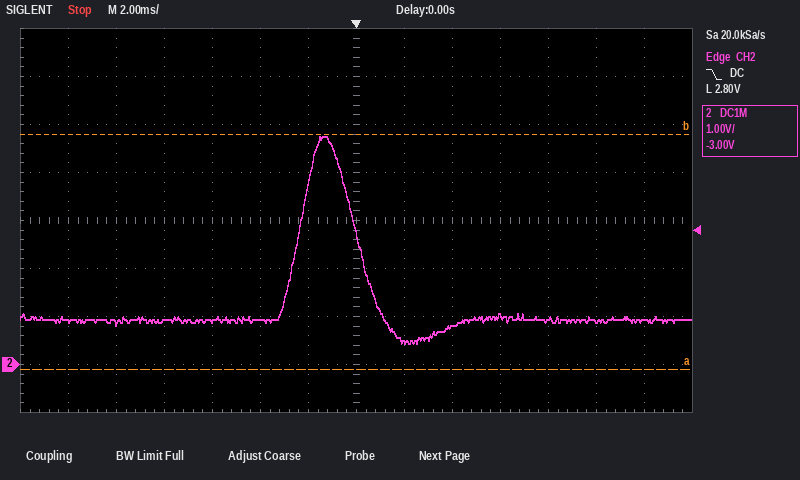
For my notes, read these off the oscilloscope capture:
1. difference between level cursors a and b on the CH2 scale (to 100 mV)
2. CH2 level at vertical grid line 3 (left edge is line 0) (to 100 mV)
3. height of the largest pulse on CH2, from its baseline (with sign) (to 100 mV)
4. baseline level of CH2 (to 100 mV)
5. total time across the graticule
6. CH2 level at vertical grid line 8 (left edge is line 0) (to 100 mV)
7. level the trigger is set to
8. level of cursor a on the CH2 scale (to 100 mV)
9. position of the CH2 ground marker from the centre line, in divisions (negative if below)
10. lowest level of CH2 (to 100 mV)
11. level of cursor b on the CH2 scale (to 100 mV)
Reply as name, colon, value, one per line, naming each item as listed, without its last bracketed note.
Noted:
difference between level cursors a and b on the CH2 scale: 4.9 V
CH2 level at vertical grid line 3 (left edge is line 0): 900 mV
height of the largest pulse on CH2, from its baseline (with sign): +3.8 V
baseline level of CH2: 900 mV
total time across the graticule: 28 ms
CH2 level at vertical grid line 8 (left edge is line 0): 500 mV
level the trigger is set to: 2.80 V
level of cursor a on the CH2 scale: -100 mV
position of the CH2 ground marker from the centre line, in divisions: -3.0 div
lowest level of CH2: 400 mV
level of cursor b on the CH2 scale: 4.8 V
